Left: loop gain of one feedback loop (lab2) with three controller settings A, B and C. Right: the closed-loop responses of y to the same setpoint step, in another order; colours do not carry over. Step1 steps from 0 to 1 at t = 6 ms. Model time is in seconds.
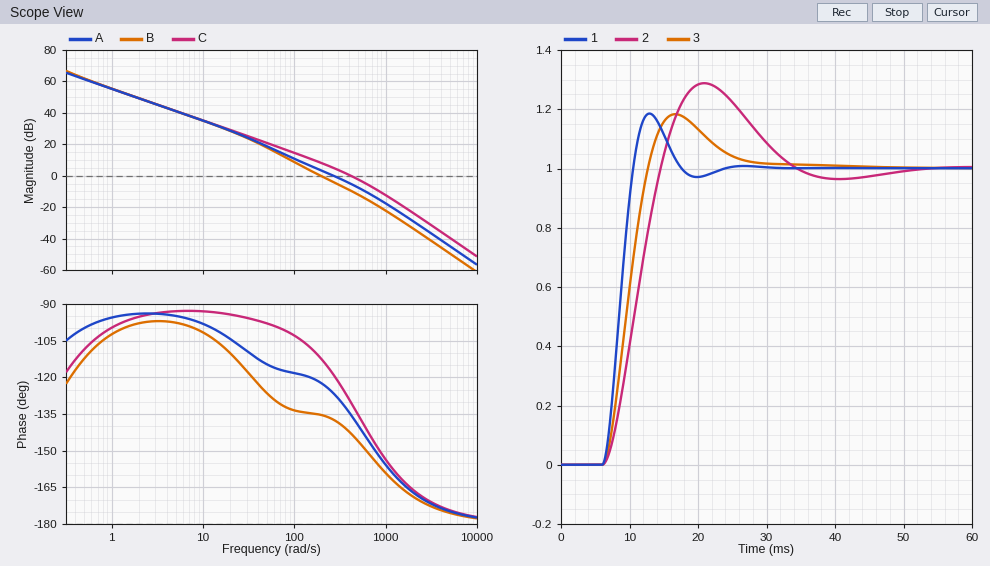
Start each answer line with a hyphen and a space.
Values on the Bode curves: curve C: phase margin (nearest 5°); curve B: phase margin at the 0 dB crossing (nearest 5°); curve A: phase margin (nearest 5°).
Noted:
- 50°
- 45°
- 55°
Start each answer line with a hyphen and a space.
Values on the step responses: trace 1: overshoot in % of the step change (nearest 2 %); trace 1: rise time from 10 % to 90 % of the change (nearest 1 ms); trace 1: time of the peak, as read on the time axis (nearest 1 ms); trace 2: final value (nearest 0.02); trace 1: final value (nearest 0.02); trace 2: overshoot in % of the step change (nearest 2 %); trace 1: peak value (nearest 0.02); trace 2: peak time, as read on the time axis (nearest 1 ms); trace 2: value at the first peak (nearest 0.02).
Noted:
- 18 %
- 3 ms
- 13 ms
- 1.00
- 1.00
- 28 %
- 1.18
- 21 ms
- 1.28
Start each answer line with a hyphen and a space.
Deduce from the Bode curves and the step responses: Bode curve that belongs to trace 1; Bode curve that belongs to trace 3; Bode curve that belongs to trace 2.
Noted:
- C
- A
- B
